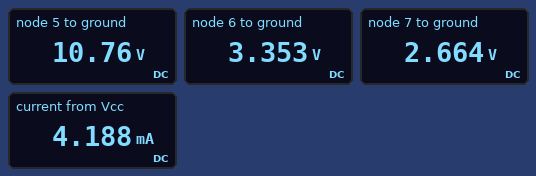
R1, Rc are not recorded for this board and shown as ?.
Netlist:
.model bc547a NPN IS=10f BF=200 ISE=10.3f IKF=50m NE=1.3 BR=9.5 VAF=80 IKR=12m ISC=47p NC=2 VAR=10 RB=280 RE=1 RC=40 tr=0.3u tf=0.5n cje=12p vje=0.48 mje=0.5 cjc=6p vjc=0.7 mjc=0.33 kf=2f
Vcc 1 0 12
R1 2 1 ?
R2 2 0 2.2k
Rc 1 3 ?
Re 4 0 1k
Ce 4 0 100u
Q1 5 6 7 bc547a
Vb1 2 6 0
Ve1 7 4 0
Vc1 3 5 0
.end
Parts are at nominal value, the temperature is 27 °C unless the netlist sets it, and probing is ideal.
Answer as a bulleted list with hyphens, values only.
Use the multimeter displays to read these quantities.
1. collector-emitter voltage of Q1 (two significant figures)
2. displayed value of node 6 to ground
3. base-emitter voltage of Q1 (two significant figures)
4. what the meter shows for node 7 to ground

- 8.1 V
- 3.353 V
- 690 mV
- 2.664 V
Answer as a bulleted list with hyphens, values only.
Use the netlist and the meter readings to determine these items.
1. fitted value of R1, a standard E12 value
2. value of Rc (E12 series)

- 5.6 kΩ
- 470 Ω
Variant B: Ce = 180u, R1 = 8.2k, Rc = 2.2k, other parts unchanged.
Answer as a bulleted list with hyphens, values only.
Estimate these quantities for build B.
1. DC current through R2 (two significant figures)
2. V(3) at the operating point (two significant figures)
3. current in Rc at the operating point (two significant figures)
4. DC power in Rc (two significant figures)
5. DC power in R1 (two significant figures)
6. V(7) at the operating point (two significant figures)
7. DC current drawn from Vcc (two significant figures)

- 1.1 mA
- 8.0 V
- 1.8 mA
- 7.3 mW
- 11 mW
- 1.8 V
- 3.0 mA
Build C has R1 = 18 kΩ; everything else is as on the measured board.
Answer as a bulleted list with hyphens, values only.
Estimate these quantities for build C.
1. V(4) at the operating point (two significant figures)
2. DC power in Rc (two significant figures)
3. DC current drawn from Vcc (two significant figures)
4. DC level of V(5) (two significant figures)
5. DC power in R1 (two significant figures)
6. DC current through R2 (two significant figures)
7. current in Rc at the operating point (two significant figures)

- 650 mV
- 200 µW
- 1.2 mA
- 12 V
- 6.4 mW
- 590 µA
- 650 µA
